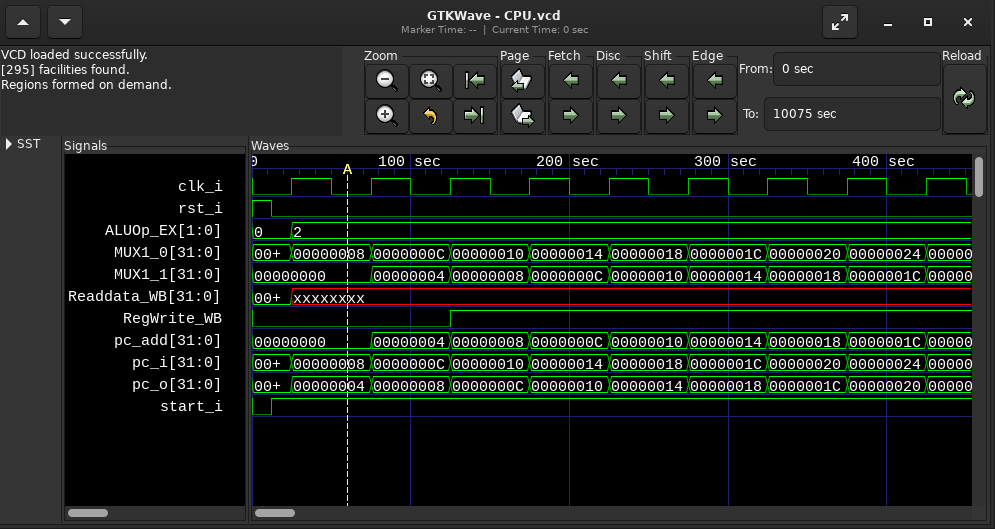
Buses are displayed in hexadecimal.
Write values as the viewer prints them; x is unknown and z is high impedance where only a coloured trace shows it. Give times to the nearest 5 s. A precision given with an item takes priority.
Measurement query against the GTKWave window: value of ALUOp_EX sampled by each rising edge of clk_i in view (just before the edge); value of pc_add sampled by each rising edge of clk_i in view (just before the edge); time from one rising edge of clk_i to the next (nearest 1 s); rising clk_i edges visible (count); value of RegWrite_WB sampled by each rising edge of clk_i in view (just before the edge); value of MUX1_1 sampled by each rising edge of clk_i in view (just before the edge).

0, 2, 2, 2, 2, 2, 2, 2, 2
00000000, 00000000, 00000004, 00000008, 0000000C, 00000010, 00000014, 00000018, 0000001C
50 s
9
0 0 0 1 1 1 1 1 1
00000000, 00000000, 00000004, 00000008, 0000000C, 00000010, 00000014, 00000018, 0000001C
